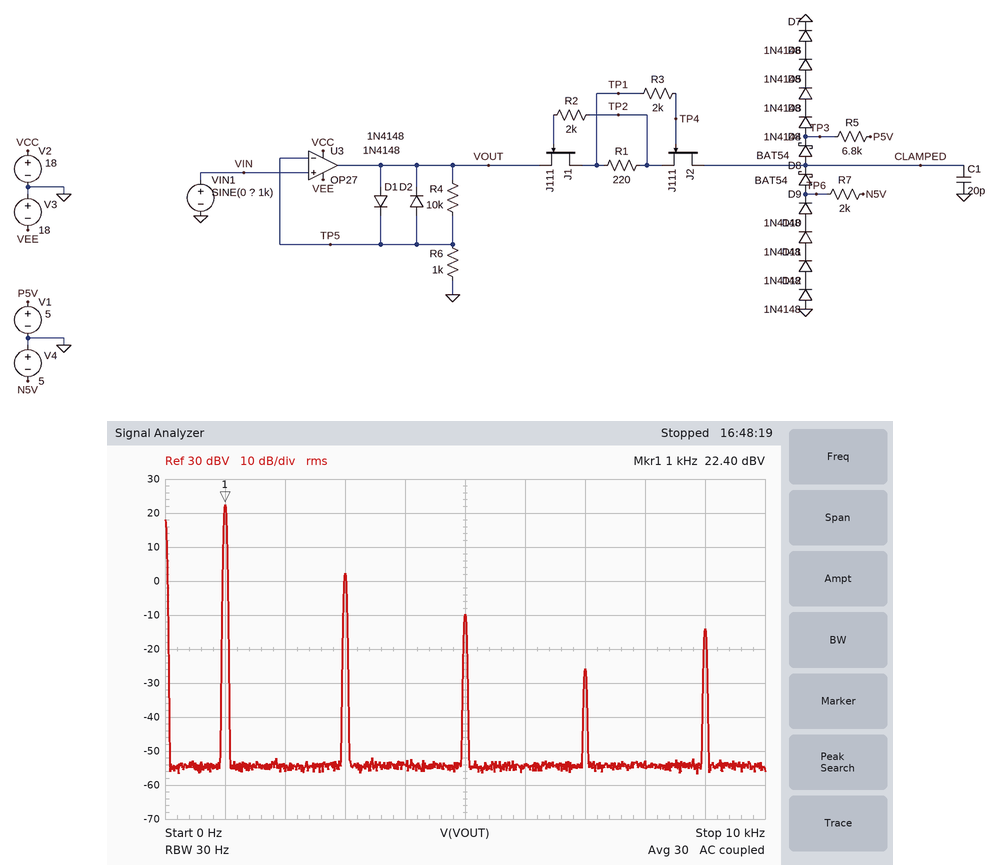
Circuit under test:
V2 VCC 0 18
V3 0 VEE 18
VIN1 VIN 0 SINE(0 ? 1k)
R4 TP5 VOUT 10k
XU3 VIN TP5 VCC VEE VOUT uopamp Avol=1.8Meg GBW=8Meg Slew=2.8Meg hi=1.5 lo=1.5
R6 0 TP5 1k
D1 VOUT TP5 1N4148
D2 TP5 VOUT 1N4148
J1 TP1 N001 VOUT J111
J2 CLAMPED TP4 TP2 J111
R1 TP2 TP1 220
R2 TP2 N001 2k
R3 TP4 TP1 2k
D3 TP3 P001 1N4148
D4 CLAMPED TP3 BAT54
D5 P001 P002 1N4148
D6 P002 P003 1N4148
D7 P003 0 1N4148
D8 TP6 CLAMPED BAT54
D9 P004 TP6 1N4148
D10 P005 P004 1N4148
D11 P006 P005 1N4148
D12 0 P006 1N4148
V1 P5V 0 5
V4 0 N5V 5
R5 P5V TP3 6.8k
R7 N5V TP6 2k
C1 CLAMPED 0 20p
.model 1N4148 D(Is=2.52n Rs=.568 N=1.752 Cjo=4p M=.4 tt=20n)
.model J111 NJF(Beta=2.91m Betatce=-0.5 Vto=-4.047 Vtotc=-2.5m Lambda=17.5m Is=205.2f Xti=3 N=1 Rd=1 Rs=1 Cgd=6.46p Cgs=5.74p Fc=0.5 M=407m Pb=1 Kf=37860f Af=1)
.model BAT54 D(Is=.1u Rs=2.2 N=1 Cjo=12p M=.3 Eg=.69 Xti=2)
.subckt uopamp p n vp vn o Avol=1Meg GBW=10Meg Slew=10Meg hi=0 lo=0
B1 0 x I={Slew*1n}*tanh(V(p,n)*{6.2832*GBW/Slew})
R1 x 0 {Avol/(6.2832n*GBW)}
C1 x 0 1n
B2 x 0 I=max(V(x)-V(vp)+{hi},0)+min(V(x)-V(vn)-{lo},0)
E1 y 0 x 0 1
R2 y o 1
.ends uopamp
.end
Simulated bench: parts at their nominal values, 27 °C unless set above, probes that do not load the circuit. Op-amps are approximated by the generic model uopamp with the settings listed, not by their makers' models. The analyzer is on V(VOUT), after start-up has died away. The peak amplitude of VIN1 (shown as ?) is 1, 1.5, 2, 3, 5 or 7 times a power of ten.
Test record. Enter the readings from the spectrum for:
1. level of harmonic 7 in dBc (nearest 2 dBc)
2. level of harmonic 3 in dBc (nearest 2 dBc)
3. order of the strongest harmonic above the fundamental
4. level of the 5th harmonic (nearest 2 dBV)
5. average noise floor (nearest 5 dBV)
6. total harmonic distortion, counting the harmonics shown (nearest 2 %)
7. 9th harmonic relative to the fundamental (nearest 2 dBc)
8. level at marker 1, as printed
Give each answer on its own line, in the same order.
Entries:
-48 dBc
-20 dBc
3
-10 dBV
-55 dBV
10 %
-36 dBc
22.40 dBV
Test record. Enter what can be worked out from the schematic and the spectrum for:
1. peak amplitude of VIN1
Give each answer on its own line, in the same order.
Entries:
20 V
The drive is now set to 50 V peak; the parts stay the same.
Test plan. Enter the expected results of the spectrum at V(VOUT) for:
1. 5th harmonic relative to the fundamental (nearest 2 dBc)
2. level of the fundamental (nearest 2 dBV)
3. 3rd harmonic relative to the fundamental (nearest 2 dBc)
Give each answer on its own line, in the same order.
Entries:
-18 dBc
24 dBV
-10 dBc
